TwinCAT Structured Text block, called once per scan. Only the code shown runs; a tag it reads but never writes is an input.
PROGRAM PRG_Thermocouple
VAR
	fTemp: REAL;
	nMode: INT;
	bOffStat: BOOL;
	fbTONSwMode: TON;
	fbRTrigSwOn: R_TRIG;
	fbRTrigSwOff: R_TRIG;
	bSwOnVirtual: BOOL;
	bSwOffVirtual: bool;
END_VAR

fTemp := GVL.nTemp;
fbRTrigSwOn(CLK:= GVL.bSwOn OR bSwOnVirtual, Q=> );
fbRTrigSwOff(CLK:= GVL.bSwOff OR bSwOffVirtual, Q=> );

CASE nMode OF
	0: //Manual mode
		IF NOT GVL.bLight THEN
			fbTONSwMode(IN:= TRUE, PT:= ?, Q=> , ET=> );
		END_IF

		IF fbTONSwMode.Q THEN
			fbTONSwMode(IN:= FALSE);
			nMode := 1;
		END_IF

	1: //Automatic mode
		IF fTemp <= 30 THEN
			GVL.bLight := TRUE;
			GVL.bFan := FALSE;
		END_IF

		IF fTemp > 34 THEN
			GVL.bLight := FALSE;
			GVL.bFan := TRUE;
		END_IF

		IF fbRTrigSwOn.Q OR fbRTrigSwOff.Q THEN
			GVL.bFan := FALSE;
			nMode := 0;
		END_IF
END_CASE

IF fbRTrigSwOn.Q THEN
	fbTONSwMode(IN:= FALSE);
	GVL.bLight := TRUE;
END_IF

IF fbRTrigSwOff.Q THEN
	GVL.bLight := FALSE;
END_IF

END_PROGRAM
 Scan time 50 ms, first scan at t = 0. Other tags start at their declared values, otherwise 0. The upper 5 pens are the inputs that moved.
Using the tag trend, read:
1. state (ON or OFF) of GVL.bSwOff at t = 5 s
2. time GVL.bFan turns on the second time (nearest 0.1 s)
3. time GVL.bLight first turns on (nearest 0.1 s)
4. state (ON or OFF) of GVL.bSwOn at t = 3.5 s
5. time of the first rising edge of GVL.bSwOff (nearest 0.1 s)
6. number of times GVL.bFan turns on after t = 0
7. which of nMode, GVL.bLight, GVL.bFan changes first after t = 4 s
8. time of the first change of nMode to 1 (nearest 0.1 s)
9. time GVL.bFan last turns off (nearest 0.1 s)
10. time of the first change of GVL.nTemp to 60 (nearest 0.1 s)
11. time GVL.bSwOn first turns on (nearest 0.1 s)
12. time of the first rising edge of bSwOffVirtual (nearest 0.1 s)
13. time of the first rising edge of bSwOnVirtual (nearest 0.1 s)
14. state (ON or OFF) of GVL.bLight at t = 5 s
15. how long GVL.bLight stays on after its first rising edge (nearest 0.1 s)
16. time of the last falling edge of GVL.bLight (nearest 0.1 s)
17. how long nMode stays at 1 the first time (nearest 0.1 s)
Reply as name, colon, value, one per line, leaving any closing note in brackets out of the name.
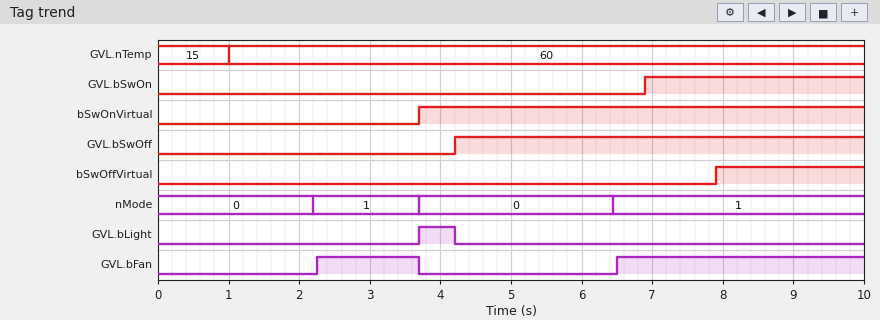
state (ON or OFF) of GVL.bSwOff at t = 5 s: ON
time GVL.bFan turns on the second time: 6.5 s
time GVL.bLight first turns on: 3.7 s
state (ON or OFF) of GVL.bSwOn at t = 3.5 s: OFF
time of the first rising edge of GVL.bSwOff: 4.2 s
number of times GVL.bFan turns on after t = 0: 2
which of nMode, GVL.bLight, GVL.bFan changes first after t = 4 s: GVL.bLight
time of the first change of nMode to 1: 2.2 s
time GVL.bFan last turns off: 3.7 s
time of the first change of GVL.nTemp to 60: 1.0 s
time GVL.bSwOn first turns on: 6.9 s
time of the first rising edge of bSwOffVirtual: 7.9 s
time of the first rising edge of bSwOnVirtual: 3.7 s
state (ON or OFF) of GVL.bLight at t = 5 s: OFF
how long GVL.bLight stays on after its first rising edge: 0.5 s
time of the last falling edge of GVL.bLight: 4.2 s
how long nMode stays at 1 the first time: 1.5 s
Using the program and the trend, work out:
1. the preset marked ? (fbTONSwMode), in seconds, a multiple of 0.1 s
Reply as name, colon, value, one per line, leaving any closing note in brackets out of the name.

the preset marked ? (fbTONSwMode), in seconds, a multiple of 0.1 s: 2.2 s
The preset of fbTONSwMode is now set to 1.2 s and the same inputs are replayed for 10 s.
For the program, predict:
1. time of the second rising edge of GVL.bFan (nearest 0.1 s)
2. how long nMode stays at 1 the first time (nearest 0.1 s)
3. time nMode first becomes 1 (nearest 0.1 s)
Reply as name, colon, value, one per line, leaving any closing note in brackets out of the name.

time of the second rising edge of GVL.bFan: 5.5 s
how long nMode stays at 1 the first time: 2.5 s
time nMode first becomes 1: 1.2 s
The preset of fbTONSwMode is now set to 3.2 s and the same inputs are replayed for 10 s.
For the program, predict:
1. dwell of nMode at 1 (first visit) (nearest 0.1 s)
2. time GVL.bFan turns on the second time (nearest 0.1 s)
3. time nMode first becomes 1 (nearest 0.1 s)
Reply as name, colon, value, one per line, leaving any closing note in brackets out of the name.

dwell of nMode at 1 (first visit): 0.5 s
time GVL.bFan turns on the second time: 7.5 s
time nMode first becomes 1: 3.2 s
